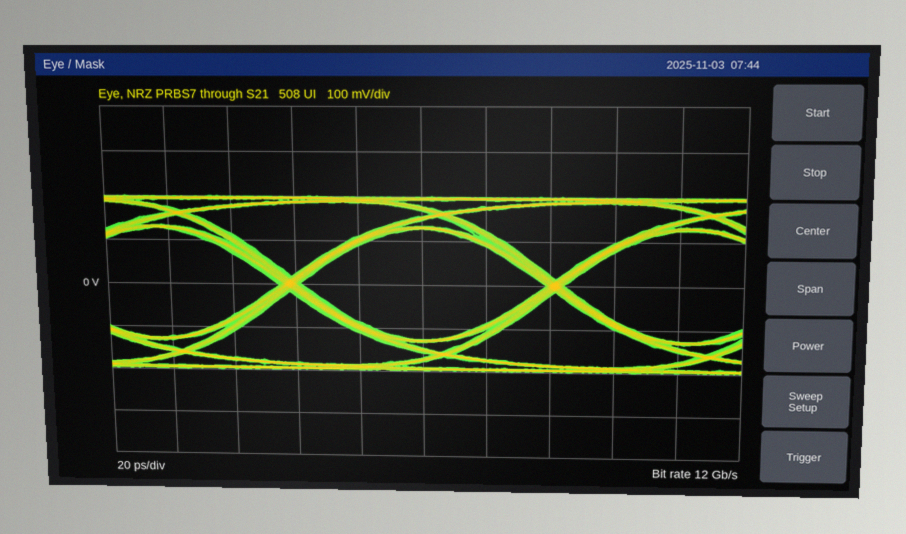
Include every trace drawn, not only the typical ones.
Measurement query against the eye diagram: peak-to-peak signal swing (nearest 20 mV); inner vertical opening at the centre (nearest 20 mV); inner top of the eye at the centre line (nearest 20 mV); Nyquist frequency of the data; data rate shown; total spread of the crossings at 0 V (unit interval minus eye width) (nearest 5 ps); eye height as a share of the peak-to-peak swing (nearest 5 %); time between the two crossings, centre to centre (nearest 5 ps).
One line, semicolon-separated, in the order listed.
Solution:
400 mV; 260 mV; 120 mV; 6 GHz; 12 Gb/s; 5 ps; 65 %; 85 ps
